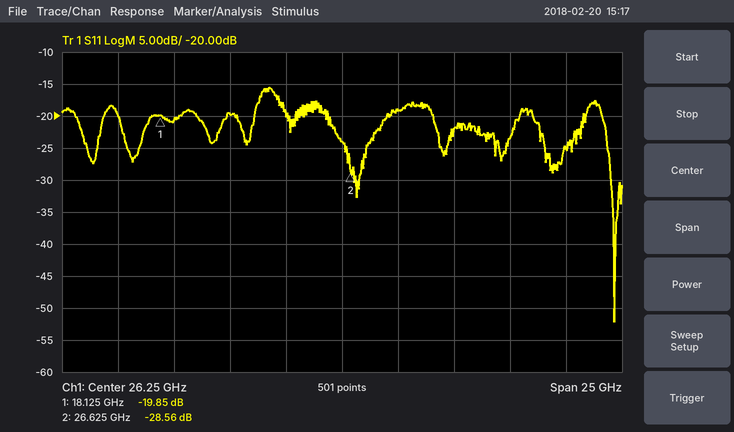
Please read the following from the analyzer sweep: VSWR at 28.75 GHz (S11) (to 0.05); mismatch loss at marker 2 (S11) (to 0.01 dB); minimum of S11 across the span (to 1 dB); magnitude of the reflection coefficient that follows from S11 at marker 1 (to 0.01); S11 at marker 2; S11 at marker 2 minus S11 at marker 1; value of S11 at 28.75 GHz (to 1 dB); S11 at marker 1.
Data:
1.25
0.01 dB
-52 dB
0.10
-28.56 dB
-8.71 dB
-19 dB
-19.85 dB
